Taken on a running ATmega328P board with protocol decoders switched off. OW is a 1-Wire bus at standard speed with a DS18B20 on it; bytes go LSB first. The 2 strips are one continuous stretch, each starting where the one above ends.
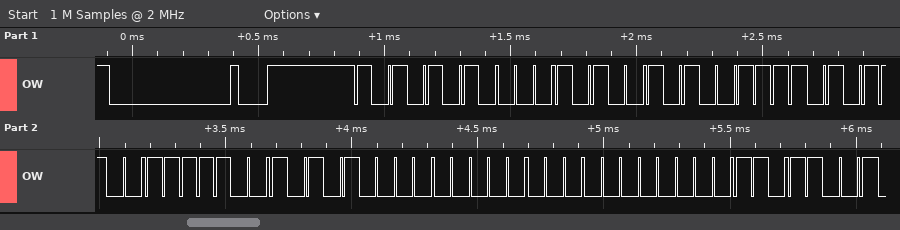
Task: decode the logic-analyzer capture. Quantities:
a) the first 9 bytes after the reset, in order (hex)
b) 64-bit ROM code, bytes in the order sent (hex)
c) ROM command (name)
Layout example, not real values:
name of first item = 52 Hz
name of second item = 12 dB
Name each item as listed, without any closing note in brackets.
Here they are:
the first 9 bytes after the reset, in order = 55 28 E5 35 9F 0A 00 00 9B
64-bit ROM code, bytes in the order sent = 28 E5 35 9F 0A 00 00 9B
ROM command = Match ROM
